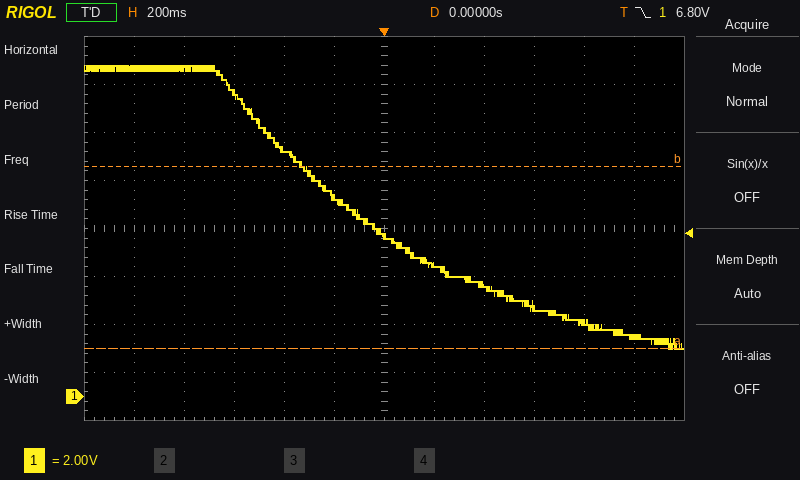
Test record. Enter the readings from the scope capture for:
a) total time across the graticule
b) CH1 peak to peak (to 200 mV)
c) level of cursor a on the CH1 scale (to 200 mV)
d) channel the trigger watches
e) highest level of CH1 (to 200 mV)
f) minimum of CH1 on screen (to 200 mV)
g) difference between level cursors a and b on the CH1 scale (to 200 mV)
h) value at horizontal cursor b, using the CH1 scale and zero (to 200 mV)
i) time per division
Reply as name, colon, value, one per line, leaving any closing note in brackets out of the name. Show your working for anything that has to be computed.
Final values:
total time across the graticule: 2.4 s
CH1 peak to peak: 13.8 V − (2.0 V) = 11.8 V
level of cursor a on the CH1 scale: 2.0 V
channel the trigger watches: CH1
highest level of CH1: 13.8 V
minimum of CH1 on screen: 2.0 V
difference between level cursors a and b on the CH1 scale: 7.6 V
value at horizontal cursor b, using the CH1 scale and zero: 9.6 V
time per division: 200 ms
